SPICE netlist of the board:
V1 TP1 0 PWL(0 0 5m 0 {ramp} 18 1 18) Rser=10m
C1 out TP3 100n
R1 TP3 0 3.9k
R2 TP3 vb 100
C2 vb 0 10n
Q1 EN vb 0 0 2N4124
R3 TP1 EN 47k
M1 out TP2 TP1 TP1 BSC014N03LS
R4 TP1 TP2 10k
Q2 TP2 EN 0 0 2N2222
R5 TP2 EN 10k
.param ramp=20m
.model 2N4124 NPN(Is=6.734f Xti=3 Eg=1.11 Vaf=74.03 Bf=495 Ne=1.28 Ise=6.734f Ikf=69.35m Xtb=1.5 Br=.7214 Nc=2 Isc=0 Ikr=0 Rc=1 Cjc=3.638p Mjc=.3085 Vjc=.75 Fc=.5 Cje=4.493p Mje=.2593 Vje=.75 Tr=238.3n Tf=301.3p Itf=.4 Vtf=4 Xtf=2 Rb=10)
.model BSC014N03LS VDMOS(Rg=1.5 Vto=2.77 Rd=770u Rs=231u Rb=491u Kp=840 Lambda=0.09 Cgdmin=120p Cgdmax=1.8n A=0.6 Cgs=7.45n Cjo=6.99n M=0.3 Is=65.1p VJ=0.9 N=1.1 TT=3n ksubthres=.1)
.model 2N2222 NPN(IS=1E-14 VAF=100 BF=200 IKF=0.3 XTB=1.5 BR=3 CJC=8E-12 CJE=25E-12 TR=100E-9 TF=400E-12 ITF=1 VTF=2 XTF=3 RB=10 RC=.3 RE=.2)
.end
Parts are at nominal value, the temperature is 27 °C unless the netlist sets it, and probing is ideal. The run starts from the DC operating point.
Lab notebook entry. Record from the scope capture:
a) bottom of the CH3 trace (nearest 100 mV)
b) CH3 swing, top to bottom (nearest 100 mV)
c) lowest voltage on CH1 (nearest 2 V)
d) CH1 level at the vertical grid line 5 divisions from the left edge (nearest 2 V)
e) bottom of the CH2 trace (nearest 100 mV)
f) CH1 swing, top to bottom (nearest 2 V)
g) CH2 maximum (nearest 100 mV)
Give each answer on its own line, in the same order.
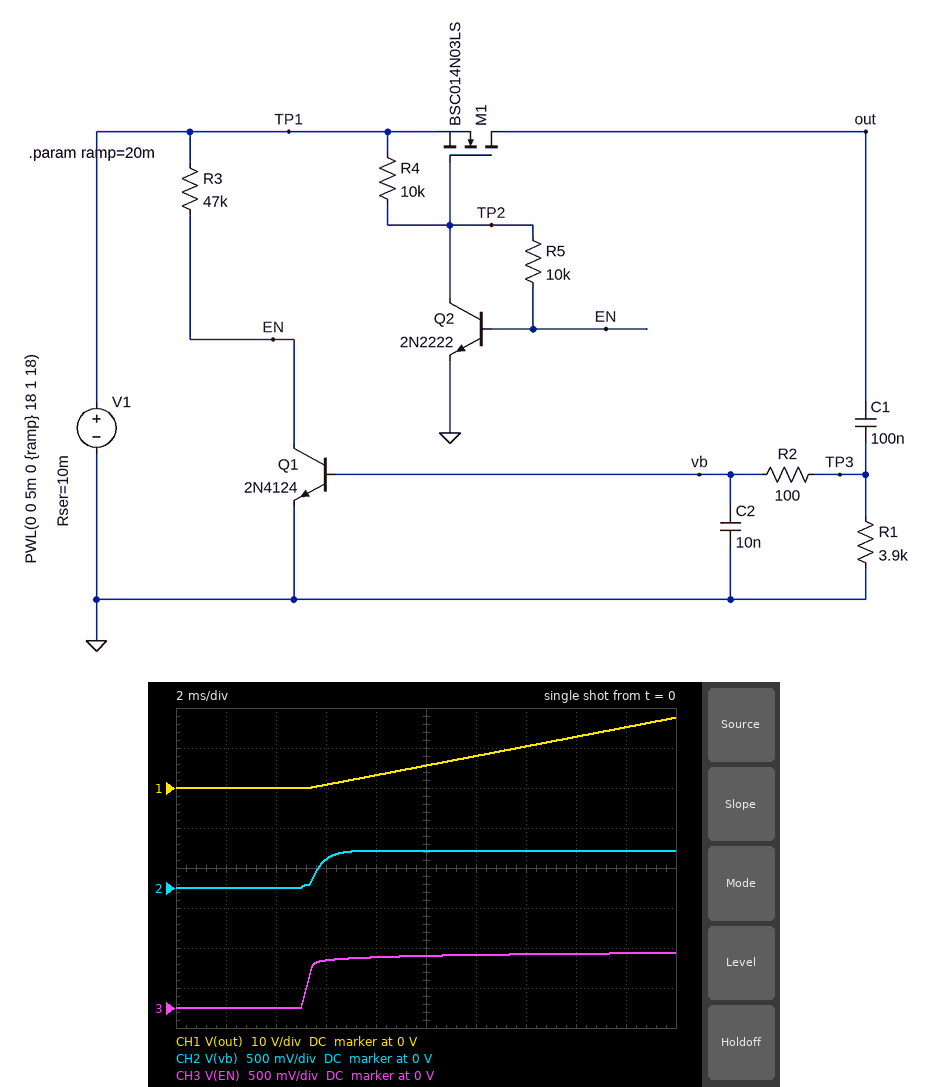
0 V
700 mV
0 V
6 V
0 V
18 V
500 mV
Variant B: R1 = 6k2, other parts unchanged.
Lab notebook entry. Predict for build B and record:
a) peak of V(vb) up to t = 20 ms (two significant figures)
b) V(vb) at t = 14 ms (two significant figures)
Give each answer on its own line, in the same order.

670 mV
660 mV
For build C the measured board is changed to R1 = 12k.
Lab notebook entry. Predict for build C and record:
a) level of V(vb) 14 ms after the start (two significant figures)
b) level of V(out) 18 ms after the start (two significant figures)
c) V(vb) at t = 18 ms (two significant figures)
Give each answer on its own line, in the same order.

660 mV
15 V
670 mV
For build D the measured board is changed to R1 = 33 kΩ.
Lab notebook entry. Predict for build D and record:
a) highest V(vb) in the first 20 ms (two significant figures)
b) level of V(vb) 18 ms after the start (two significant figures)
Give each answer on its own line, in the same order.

680 mV
670 mV
